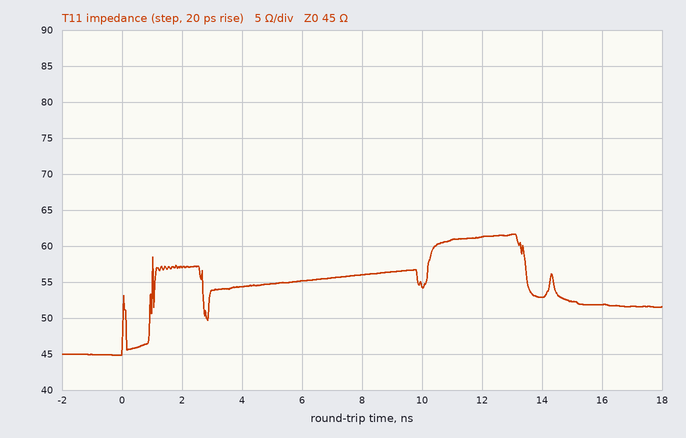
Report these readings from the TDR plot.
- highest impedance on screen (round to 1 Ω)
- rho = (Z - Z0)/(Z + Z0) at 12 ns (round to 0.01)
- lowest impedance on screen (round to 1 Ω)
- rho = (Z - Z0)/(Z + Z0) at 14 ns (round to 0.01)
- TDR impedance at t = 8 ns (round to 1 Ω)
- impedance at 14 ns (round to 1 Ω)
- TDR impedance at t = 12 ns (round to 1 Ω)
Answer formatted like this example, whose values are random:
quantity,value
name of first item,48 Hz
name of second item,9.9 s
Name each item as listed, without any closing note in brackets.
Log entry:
quantity,value
highest impedance on screen,62 Ω
rho = (Z - Z0)/(Z + Z0) at 12 ns,+0.15
lowest impedance on screen,45 Ω
rho = (Z - Z0)/(Z + Z0) at 14 ns,+0.08
TDR impedance at t = 8 ns,56 Ω
impedance at 14 ns,53 Ω
TDR impedance at t = 12 ns,61 Ω
